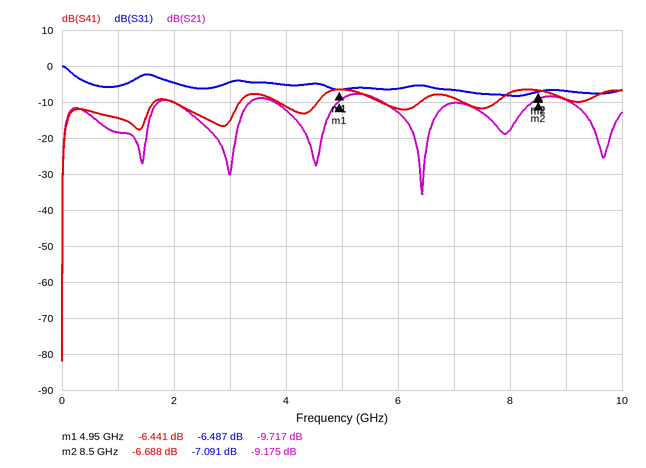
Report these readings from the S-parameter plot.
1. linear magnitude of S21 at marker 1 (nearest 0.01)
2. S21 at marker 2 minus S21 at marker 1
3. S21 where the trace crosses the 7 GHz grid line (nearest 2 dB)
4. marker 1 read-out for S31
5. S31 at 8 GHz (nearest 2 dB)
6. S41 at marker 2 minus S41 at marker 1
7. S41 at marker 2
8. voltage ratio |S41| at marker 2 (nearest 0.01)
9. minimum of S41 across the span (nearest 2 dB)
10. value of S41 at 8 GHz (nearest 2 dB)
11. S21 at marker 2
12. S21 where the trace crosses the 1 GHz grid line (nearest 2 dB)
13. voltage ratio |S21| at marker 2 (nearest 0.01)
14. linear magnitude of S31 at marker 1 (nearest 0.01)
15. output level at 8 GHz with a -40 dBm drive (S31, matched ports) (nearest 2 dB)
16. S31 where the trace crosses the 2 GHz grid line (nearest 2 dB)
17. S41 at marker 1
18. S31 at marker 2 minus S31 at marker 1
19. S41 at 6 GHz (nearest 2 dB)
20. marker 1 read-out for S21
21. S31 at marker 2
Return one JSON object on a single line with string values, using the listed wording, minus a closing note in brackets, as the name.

{"linear magnitude of S21 at marker 1": "0.33", "S21 at marker 2 minus S21 at marker 1": "0.542 dB", "S21 where the trace crosses the 7 GHz grid line": "-10 dB", "marker 1 read-out for S31": "-6.487 dB", "S31 at 8 GHz": "-8 dB", "S41 at marker 2 minus S41 at marker 1": "-0.247 dB", "S41 at marker 2": "-6.688 dB", "voltage ratio |S41| at marker 2": "0.46", "minimum of S41 across the span": "-82 dB", "value of S41 at 8 GHz": "-8 dB", "S21 at marker 2": "-9.175 dB", "S21 where the trace crosses the 1 GHz grid line": "-18 dB", "voltage ratio |S21| at marker 2": "0.35", "linear magnitude of S31 at marker 1": "0.47", "output level at 8 GHz with a -40 dBm drive (S31, matched ports)": "-48 dBm", "S31 where the trace crosses the 2 GHz grid line": "-4 dB", "S41 at marker 1": "-6.441 dB", "S31 at marker 2 minus S31 at marker 1": "-0.604 dB", "S41 at 6 GHz": "-12 dB", "marker 1 read-out for S21": "-9.717 dB", "S31 at marker 2": "-7.091 dB"}
